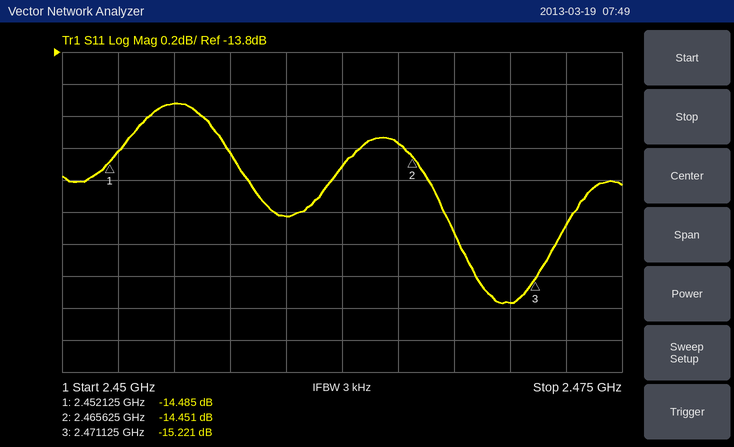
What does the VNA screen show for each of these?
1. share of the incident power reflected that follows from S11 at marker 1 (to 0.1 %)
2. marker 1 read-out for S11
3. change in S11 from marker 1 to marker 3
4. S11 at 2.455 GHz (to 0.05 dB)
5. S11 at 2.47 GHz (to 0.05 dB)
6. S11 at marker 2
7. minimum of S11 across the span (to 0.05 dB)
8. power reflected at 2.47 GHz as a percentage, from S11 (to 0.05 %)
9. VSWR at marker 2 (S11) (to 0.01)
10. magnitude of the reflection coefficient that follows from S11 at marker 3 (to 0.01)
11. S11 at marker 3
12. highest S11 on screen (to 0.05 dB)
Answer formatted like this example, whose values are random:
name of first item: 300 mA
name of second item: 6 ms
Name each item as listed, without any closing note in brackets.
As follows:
share of the incident power reflected that follows from S11 at marker 1: 3.6 %
marker 1 read-out for S11: -14.485 dB
change in S11 from marker 1 to marker 3: -0.736 dB
S11 at 2.455 GHz: -14.10 dB
S11 at 2.47 GHz: -15.35 dB
S11 at marker 2: -14.451 dB
minimum of S11 across the span: -15.35 dB
power reflected at 2.47 GHz as a percentage, from S11: 2.90 %
VSWR at marker 2 (S11): 1.47
magnitude of the reflection coefficient that follows from S11 at marker 3: 0.17
S11 at marker 3: -15.221 dB
highest S11 on screen: -14.10 dB
